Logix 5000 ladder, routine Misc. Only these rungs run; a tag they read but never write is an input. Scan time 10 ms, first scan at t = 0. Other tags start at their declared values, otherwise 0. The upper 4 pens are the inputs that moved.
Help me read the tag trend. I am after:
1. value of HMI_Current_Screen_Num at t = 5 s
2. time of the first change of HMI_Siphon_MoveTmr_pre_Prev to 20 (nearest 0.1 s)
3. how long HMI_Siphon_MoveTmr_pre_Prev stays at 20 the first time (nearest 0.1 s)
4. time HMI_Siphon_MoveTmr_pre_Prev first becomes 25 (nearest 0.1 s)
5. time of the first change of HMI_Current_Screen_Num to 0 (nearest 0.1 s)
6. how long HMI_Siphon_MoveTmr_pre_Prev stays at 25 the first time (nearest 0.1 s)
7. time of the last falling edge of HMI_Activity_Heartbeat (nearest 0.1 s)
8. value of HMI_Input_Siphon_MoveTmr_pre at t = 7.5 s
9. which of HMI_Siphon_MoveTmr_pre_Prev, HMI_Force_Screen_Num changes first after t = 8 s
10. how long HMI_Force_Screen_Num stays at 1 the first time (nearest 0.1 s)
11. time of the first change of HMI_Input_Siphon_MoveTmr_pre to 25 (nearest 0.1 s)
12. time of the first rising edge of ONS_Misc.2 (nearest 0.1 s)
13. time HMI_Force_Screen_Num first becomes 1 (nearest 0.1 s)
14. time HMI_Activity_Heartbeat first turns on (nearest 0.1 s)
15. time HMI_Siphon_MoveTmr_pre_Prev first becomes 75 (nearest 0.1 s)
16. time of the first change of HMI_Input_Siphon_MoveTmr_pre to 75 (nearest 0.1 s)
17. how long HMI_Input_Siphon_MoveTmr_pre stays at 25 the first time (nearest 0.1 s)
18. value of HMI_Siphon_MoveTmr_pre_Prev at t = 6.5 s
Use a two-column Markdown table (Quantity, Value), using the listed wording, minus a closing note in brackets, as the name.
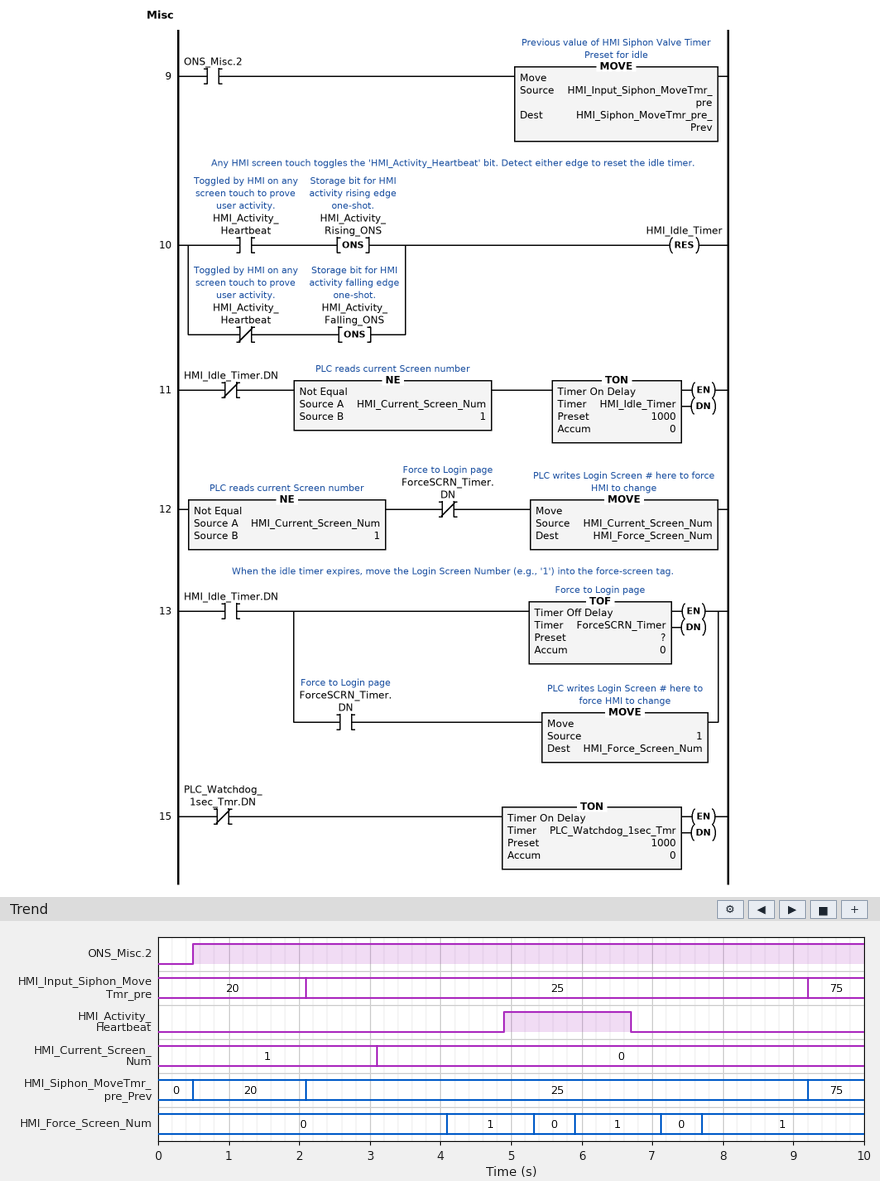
| Quantity | Value |
|---|---|
| value of HMI_Current_Screen_Num at t = 5 s | 0 |
| time of the first change of HMI_Siphon_MoveTmr_pre_Prev to 20 | 0.5 s |
| how long HMI_Siphon_MoveTmr_pre_Prev stays at 20 the first time | 1.6 s |
| time HMI_Siphon_MoveTmr_pre_Prev first becomes 25 | 2.1 s |
| time of the first change of HMI_Current_Screen_Num to 0 | 3.1 s |
| how long HMI_Siphon_MoveTmr_pre_Prev stays at 25 the first time | 7.1 s |
| time of the last falling edge of HMI_Activity_Heartbeat | 6.7 s |
| value of HMI_Input_Siphon_MoveTmr_pre at t = 7.5 s | 25 |
| which of HMI_Siphon_MoveTmr_pre_Prev, HMI_Force_Screen_Num changes first after t = 8 s | HMI_Siphon_MoveTmr_pre_Prev |
| how long HMI_Force_Screen_Num stays at 1 the first time | 1.2 s |
| time of the first change of HMI_Input_Siphon_MoveTmr_pre to 25 | 2.1 s |
| time of the first rising edge of ONS_Misc.2 | 0.5 s |
| time HMI_Force_Screen_Num first becomes 1 | 4.1 s |
| time HMI_Activity_Heartbeat first turns on | 4.9 s |
| time HMI_Siphon_MoveTmr_pre_Prev first becomes 75 | 9.2 s |
| time of the first change of HMI_Input_Siphon_MoveTmr_pre to 75 | 9.2 s |
| how long HMI_Input_Siphon_MoveTmr_pre stays at 25 the first time | 7.1 s |
| value of HMI_Siphon_MoveTmr_pre_Prev at t = 6.5 s | 25 |
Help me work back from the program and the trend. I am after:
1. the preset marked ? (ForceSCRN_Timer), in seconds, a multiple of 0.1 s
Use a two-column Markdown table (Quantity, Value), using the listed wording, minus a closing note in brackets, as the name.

| Quantity | Value |
|---|---|
| the preset marked ? (ForceSCRN_Timer), in seconds, a multiple of 0.1 s | 1.2 s |
